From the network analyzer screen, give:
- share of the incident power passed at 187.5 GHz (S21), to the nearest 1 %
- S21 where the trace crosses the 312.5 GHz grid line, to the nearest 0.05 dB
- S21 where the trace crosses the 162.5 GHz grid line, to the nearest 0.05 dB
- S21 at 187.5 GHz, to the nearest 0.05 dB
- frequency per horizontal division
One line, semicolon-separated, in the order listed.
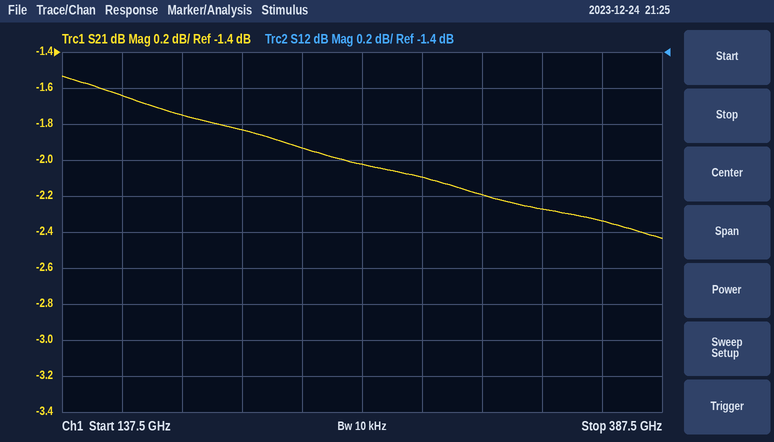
67 %; -2.20 dB; -1.65 dB; -1.75 dB; 25 GHz
